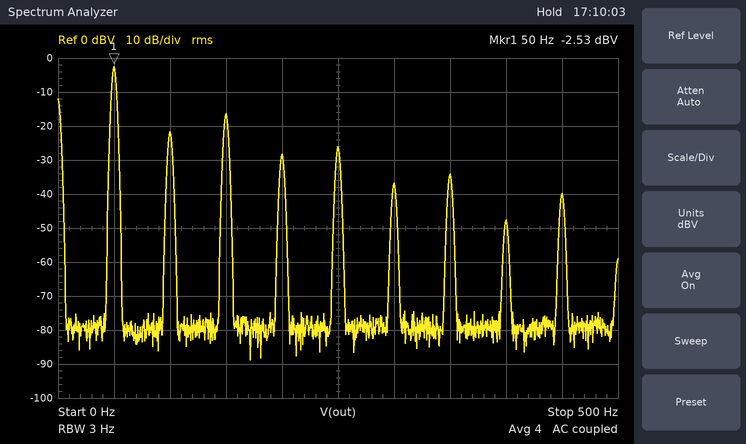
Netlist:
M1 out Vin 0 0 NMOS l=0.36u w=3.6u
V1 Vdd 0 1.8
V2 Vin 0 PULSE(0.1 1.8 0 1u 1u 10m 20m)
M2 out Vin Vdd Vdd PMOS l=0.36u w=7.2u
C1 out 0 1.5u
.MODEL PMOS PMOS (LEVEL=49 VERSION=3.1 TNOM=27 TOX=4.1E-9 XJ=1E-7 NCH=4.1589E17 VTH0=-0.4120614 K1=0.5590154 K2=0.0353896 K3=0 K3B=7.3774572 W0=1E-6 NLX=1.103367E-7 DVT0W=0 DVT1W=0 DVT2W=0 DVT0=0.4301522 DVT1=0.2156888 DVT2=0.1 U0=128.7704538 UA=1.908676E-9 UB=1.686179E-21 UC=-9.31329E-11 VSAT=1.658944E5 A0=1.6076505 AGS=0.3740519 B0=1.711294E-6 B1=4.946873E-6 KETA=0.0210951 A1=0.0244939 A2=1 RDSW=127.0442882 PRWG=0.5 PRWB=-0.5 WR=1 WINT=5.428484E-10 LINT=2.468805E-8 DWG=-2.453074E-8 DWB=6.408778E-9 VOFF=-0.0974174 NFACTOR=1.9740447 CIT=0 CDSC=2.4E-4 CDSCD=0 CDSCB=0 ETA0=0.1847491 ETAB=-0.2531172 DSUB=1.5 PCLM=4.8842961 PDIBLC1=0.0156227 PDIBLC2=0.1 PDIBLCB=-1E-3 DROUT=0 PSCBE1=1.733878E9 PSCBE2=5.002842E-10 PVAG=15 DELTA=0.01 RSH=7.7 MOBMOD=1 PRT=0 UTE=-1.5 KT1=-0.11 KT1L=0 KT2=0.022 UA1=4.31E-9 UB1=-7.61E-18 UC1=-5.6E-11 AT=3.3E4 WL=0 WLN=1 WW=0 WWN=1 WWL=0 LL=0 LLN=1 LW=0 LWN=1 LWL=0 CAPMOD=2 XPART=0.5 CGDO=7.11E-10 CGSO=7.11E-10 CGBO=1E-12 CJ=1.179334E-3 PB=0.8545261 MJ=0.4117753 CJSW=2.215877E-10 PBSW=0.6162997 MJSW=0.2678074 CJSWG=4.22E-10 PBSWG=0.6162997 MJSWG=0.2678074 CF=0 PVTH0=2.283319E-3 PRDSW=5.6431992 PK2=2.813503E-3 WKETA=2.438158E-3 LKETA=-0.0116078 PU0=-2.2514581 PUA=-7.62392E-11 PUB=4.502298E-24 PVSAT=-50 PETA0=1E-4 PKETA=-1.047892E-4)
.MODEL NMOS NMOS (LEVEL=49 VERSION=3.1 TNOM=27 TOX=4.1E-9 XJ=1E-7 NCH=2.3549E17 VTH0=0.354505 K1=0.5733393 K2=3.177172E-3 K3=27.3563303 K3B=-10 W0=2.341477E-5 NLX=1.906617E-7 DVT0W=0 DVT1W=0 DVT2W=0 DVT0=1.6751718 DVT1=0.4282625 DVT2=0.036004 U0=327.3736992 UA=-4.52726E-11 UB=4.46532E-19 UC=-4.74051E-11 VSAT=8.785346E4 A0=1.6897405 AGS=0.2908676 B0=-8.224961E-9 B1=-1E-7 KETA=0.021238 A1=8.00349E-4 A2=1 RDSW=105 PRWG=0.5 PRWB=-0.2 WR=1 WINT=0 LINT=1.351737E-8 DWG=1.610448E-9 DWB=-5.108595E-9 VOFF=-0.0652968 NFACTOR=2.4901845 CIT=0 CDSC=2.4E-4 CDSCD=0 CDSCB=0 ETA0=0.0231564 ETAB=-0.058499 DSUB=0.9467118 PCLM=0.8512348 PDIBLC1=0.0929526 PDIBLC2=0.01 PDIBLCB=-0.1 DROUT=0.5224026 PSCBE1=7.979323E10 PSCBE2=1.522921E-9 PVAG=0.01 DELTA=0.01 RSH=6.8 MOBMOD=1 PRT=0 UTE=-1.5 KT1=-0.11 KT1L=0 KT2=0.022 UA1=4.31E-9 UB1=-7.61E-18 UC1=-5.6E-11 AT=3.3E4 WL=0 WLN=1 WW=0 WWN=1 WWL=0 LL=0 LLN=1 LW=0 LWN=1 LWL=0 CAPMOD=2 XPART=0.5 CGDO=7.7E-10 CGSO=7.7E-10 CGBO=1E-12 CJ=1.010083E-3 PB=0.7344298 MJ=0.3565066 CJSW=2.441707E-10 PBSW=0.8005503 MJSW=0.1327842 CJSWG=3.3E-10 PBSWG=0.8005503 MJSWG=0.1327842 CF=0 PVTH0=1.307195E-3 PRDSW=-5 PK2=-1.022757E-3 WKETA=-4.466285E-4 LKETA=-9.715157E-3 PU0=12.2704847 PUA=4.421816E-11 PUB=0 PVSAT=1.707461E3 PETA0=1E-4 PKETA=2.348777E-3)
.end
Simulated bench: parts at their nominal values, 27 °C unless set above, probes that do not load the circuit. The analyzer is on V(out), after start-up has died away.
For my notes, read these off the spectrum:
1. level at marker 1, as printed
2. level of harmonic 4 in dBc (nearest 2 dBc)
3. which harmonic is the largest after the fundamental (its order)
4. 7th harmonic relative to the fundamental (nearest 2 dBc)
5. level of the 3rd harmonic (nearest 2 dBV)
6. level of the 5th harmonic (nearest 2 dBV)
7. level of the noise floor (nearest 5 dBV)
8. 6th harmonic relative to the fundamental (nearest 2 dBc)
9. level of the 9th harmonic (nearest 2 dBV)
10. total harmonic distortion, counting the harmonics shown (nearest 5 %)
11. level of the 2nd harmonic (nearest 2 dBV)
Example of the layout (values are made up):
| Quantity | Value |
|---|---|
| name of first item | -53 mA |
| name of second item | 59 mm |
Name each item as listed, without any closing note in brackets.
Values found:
| Quantity | Value |
|---|---|
| level at marker 1, as printed | -2.53 dBV |
| level of harmonic 4 in dBc | -26 dBc |
| which harmonic is the largest after the fundamental | 3 |
| 7th harmonic relative to the fundamental | -32 dBc |
| level of the 3rd harmonic | -16 dBV |
| level of the 5th harmonic | -26 dBV |
| level of the noise floor | -80 dBV |
| 6th harmonic relative to the fundamental | -34 dBc |
| level of the 9th harmonic | -40 dBV |
| total harmonic distortion, counting the harmonics shown | 25 % |
| level of the 2nd harmonic | -22 dBV |
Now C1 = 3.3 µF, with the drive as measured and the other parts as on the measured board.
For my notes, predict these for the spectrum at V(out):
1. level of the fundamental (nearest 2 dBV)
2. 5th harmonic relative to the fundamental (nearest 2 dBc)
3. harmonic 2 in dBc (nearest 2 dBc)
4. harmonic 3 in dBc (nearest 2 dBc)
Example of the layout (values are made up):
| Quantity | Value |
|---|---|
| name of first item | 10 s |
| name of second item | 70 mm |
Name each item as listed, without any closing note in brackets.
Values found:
| Quantity | Value |
|---|---|
| level of the fundamental | -4 dBV |
| 5th harmonic relative to the fundamental | -30 dBc |
| harmonic 2 in dBc | -18 dBc |
| harmonic 3 in dBc | -20 dBc |
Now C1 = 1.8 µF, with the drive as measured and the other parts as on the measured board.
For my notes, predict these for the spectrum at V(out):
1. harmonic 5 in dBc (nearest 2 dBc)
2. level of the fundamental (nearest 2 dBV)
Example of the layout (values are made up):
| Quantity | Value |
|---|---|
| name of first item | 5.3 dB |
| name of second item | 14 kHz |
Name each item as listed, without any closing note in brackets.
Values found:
| Quantity | Value |
|---|---|
| harmonic 5 in dBc | -26 dBc |
| level of the fundamental | -2 dBV |
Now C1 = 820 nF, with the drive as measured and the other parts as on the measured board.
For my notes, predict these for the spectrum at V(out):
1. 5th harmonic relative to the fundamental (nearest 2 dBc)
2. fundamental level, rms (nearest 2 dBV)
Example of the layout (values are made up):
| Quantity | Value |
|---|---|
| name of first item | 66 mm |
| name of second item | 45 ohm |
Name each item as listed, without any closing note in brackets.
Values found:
| Quantity | Value |
|---|---|
| 5th harmonic relative to the fundamental | -18 dBc |
| fundamental level, rms | -2 dBV |
